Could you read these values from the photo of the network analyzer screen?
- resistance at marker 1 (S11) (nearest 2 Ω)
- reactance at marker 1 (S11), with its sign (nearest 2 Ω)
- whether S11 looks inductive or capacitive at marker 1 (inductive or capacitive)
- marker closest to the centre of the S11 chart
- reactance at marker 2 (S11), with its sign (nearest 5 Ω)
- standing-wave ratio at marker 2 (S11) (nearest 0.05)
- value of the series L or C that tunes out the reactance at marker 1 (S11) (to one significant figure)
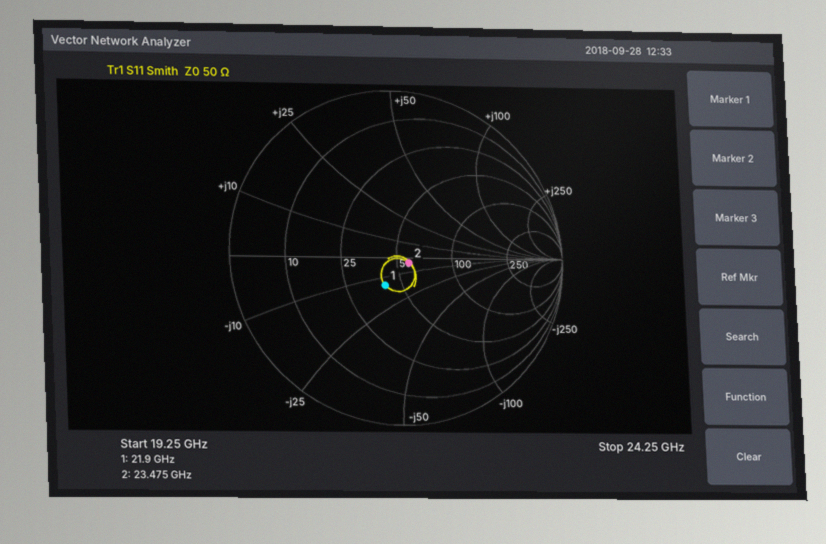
40 Ω
-14 Ω
capacitive
marker 2
-5 Ω
1.15
100 pH
